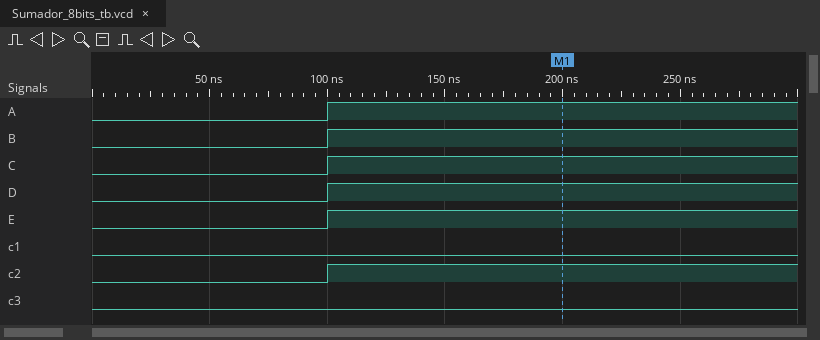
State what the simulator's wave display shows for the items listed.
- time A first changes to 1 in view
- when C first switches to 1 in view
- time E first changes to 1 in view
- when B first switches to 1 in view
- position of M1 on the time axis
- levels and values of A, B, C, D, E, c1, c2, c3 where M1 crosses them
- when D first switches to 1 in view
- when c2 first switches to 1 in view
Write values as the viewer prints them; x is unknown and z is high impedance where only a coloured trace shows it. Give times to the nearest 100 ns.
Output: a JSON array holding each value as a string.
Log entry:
["100 ns", "100 ns", "100 ns", "100 ns", "200 ns", "A=1, B=1, C=1, D=1, E=1, c1=0, c2=1, c3=0", "100 ns", "100 ns"]
